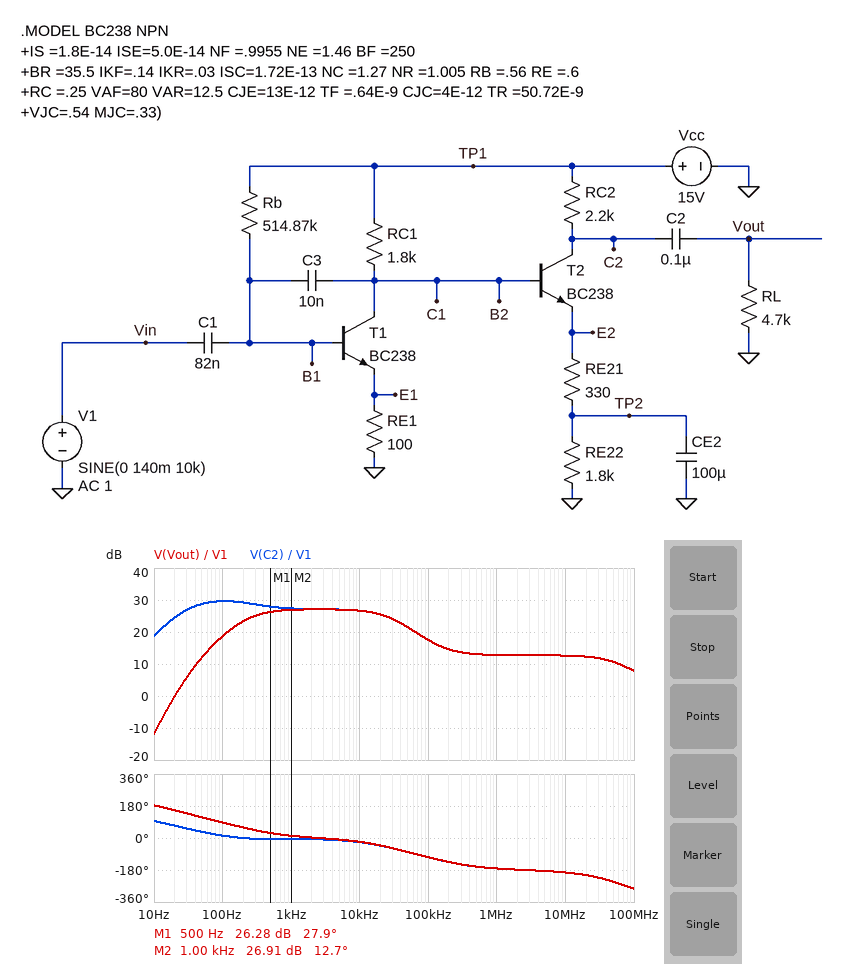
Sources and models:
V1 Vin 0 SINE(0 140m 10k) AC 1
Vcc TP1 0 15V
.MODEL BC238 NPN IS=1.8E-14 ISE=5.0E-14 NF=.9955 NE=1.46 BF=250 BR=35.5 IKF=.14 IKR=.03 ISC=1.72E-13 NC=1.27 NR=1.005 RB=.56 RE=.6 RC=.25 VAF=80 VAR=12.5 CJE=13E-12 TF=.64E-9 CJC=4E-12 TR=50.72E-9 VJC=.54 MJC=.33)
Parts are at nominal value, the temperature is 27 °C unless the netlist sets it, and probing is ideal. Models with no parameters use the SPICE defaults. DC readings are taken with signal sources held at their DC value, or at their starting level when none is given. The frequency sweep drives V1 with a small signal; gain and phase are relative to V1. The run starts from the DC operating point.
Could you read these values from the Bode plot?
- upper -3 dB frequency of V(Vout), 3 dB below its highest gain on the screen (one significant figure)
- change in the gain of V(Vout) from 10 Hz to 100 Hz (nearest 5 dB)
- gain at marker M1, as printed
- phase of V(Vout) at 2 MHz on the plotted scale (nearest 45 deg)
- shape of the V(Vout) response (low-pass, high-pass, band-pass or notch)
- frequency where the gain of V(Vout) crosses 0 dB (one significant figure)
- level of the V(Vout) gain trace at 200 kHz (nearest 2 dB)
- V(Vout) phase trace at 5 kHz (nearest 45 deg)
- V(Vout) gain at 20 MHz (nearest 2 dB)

30 kHz
30 dB
26.28 dB
-180 deg
band-pass
20 Hz
14 dB
0 deg
12 dB
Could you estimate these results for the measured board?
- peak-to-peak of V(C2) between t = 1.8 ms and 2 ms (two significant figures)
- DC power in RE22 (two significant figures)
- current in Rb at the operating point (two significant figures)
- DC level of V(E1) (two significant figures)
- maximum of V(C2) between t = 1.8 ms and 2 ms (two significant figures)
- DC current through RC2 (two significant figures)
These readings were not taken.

5.9 V
7.5 mW
27 µA
560 mV
13 V
2.0 mA
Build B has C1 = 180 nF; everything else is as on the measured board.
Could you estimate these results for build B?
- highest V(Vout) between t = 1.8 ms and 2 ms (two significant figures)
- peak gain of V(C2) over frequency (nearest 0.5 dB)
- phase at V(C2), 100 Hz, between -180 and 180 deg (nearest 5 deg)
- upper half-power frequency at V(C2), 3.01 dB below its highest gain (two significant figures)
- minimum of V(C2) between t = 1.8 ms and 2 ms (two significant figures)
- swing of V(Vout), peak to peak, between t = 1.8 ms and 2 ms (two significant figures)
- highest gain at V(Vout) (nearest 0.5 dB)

3.3 V
34.0 dB
10 deg
5.0 kHz
5.9 V
7.6 V
31.0 dB
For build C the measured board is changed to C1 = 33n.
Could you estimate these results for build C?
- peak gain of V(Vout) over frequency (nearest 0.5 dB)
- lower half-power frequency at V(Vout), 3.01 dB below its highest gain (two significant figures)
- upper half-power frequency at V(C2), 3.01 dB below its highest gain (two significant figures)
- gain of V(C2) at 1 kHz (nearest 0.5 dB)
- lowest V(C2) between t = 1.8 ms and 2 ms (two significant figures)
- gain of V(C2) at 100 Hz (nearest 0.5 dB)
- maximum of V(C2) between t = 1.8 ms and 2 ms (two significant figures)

21.0 dB
240 Hz
26 kHz
21.5 dB
8.9 V
23.5 dB
12 V
